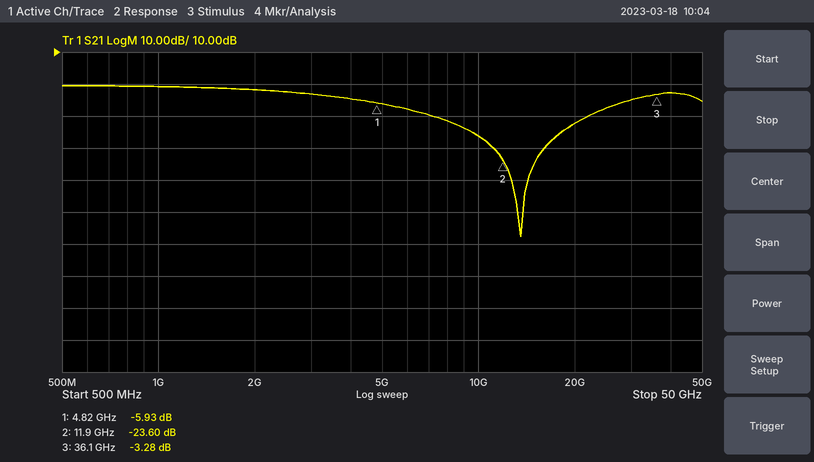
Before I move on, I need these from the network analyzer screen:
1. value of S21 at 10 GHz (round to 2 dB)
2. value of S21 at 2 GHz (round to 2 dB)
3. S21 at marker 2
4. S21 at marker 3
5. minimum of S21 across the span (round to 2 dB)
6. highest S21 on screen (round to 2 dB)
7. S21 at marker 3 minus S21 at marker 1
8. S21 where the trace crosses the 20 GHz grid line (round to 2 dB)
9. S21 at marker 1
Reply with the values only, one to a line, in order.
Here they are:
-16 dB
-2 dB
-23.60 dB
-3.28 dB
-48 dB
0 dB
2.65 dB
-12 dB
-5.93 dB
